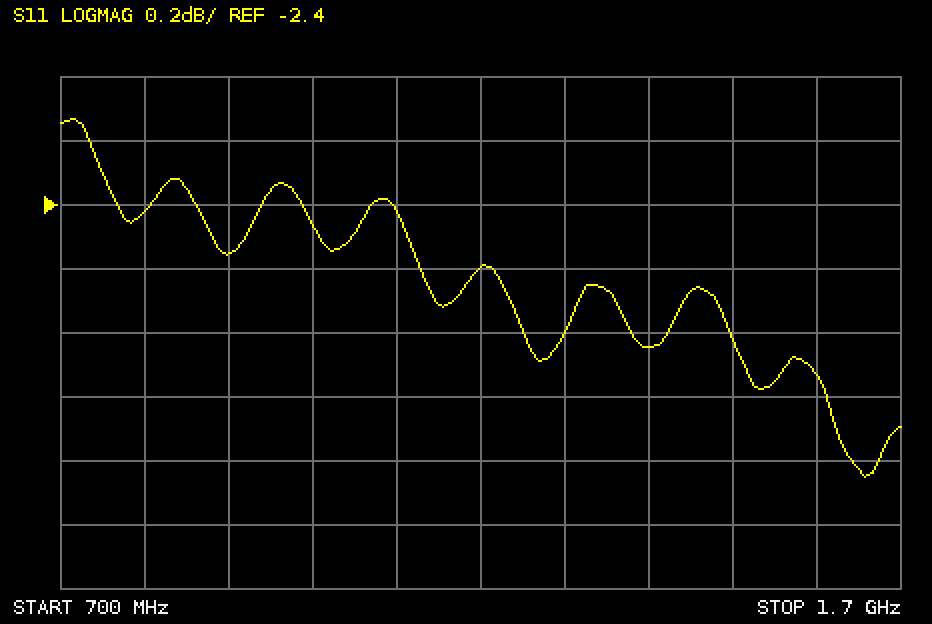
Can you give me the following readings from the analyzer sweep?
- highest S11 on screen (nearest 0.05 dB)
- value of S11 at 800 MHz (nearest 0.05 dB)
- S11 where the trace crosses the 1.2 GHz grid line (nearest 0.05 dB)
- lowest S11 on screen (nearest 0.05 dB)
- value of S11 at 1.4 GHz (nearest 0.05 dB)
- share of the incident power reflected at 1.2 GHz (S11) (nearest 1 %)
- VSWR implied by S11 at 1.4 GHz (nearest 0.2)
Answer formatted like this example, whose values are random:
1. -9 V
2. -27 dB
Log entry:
1. -2.15 dB
2. -2.40 dB
3. -2.60 dB
4. -3.25 dB
5. -2.85 dB
6. 55 %
7. 6.2
